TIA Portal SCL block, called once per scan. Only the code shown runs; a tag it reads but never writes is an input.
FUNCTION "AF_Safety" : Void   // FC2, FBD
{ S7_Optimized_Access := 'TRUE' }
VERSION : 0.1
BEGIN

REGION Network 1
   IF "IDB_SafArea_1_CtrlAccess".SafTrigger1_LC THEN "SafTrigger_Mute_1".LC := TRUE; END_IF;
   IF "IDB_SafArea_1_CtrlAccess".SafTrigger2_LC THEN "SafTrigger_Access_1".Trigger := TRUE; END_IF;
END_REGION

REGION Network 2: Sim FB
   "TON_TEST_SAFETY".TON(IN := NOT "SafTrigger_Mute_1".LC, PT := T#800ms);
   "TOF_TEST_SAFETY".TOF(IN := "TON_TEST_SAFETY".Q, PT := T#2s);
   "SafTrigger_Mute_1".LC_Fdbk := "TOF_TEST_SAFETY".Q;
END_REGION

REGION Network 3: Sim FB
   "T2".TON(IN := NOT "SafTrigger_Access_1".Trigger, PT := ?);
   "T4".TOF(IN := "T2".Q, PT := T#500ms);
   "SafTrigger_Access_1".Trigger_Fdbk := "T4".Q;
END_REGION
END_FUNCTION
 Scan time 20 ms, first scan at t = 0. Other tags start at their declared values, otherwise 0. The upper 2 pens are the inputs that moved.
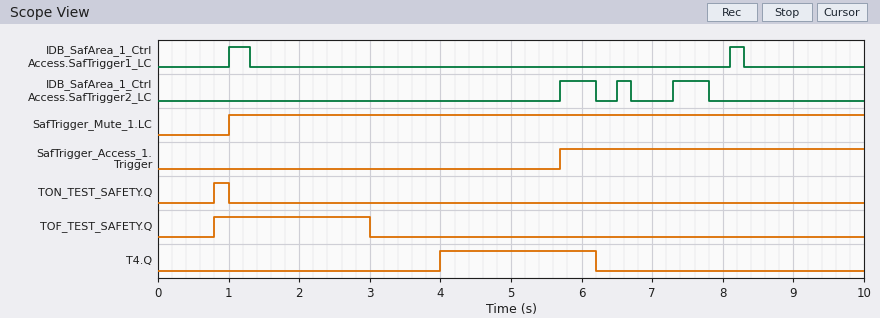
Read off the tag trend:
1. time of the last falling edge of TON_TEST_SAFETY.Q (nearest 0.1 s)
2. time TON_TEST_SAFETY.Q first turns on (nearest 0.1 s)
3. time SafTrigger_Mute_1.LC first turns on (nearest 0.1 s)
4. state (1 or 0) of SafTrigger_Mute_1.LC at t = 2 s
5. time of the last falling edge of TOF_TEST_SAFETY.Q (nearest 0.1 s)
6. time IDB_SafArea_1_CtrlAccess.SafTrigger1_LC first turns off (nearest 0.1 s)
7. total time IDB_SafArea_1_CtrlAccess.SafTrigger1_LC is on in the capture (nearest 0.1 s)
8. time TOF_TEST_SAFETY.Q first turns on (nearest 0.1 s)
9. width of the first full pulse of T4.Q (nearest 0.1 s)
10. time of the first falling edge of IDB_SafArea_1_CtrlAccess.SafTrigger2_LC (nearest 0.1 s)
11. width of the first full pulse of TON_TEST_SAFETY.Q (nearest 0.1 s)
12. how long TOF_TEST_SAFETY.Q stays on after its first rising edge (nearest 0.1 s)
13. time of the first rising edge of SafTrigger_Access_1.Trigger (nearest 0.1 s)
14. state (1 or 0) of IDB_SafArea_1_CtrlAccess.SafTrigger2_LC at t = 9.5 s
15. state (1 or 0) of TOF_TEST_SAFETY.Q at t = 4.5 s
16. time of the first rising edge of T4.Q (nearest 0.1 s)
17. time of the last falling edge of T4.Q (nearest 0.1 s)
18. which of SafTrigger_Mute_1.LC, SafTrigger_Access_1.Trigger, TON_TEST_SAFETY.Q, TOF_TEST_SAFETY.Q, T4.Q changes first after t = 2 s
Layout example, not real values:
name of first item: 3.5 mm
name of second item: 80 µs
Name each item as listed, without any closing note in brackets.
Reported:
time of the last falling edge of TON_TEST_SAFETY.Q: 1.0 s
time TON_TEST_SAFETY.Q first turns on: 0.8 s
time SafTrigger_Mute_1.LC first turns on: 1.0 s
state (1 or 0) of SafTrigger_Mute_1.LC at t = 2 s: 1
time of the last falling edge of TOF_TEST_SAFETY.Q: 3.0 s
time IDB_SafArea_1_CtrlAccess.SafTrigger1_LC first turns off: 1.3 s
total time IDB_SafArea_1_CtrlAccess.SafTrigger1_LC is on in the capture: 0.5 s
time TOF_TEST_SAFETY.Q first turns on: 0.8 s
width of the first full pulse of T4.Q: 2.2 s
time of the first falling edge of IDB_SafArea_1_CtrlAccess.SafTrigger2_LC: 6.2 s
width of the first full pulse of TON_TEST_SAFETY.Q: 0.2 s
how long TOF_TEST_SAFETY.Q stays on after its first rising edge: 2.2 s
time of the first rising edge of SafTrigger_Access_1.Trigger: 5.7 s
state (1 or 0) of IDB_SafArea_1_CtrlAccess.SafTrigger2_LC at t = 9.5 s: 0
state (1 or 0) of TOF_TEST_SAFETY.Q at t = 4.5 s: 0
time of the first rising edge of T4.Q: 4.0 s
time of the last falling edge of T4.Q: 6.2 s
which of SafTrigger_Mute_1.LC, SafTrigger_Access_1.Trigger, TON_TEST_SAFETY.Q, TOF_TEST_SAFETY.Q, T4.Q changes first after t = 2 s: TOF_TEST_SAFETY.Q
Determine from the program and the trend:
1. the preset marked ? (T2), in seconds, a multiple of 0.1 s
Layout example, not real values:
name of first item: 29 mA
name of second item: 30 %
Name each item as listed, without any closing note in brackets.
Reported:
the preset marked ? (T2), in seconds, a multiple of 0.1 s: 4.0 s
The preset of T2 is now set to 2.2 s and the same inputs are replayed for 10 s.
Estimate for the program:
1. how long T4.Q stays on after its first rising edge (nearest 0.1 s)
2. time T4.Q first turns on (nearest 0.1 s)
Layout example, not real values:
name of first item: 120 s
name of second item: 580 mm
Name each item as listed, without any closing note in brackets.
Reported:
how long T4.Q stays on after its first rising edge: 4.0 s
time T4.Q first turns on: 2.2 s
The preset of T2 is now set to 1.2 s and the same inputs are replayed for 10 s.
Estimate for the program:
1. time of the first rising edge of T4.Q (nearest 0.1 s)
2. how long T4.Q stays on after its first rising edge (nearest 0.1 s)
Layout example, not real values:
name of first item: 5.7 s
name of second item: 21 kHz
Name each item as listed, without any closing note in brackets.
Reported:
time of the first rising edge of T4.Q: 1.2 s
how long T4.Q stays on after its first rising edge: 5.0 s
